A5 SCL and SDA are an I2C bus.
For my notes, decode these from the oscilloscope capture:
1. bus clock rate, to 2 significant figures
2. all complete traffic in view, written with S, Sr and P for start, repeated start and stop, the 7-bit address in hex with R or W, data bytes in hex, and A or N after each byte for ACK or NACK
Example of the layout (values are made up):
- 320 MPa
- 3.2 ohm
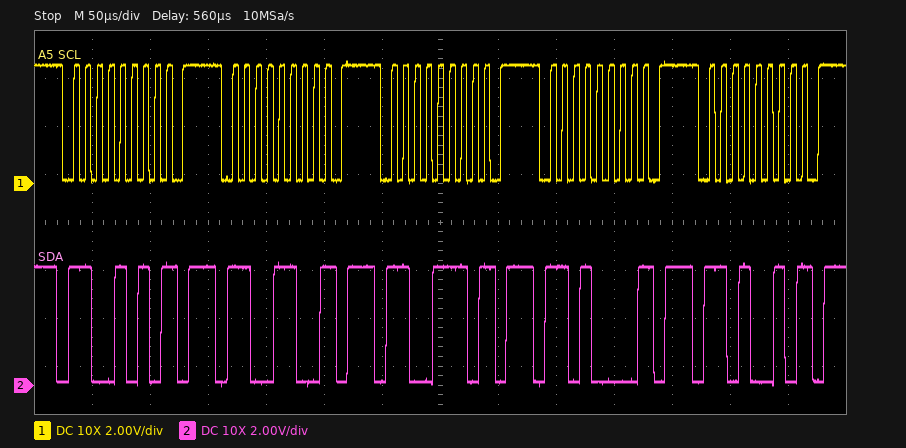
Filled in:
- 100 kHz
- S 65W N P S 66W N P S 67W N P S 68W N P S 69W N P
